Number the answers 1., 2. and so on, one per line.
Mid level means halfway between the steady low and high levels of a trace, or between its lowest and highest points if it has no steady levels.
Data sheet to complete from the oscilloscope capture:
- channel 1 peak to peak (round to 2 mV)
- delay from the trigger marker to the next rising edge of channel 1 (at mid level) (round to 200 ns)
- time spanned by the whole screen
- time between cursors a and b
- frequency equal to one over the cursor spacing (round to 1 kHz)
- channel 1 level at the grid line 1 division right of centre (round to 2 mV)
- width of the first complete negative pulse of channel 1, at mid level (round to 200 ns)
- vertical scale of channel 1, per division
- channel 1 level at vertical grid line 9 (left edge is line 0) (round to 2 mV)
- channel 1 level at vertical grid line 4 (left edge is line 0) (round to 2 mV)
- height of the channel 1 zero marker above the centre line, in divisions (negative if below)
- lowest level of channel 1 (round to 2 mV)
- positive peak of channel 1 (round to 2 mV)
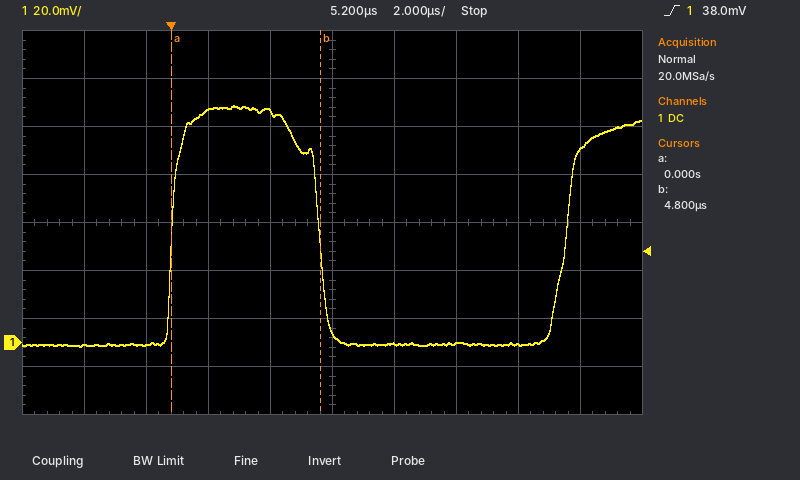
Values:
1. 100 mV
2. 12.8 µs
3. 20 µs
4. 4.8 µs
5. 208 kHz
6. 0 mV
7. 8.0 µs
8. 20 mV
9. 80 mV
10. 96 mV
11. -2.5 div
12. -2 mV
13. 98 mV
